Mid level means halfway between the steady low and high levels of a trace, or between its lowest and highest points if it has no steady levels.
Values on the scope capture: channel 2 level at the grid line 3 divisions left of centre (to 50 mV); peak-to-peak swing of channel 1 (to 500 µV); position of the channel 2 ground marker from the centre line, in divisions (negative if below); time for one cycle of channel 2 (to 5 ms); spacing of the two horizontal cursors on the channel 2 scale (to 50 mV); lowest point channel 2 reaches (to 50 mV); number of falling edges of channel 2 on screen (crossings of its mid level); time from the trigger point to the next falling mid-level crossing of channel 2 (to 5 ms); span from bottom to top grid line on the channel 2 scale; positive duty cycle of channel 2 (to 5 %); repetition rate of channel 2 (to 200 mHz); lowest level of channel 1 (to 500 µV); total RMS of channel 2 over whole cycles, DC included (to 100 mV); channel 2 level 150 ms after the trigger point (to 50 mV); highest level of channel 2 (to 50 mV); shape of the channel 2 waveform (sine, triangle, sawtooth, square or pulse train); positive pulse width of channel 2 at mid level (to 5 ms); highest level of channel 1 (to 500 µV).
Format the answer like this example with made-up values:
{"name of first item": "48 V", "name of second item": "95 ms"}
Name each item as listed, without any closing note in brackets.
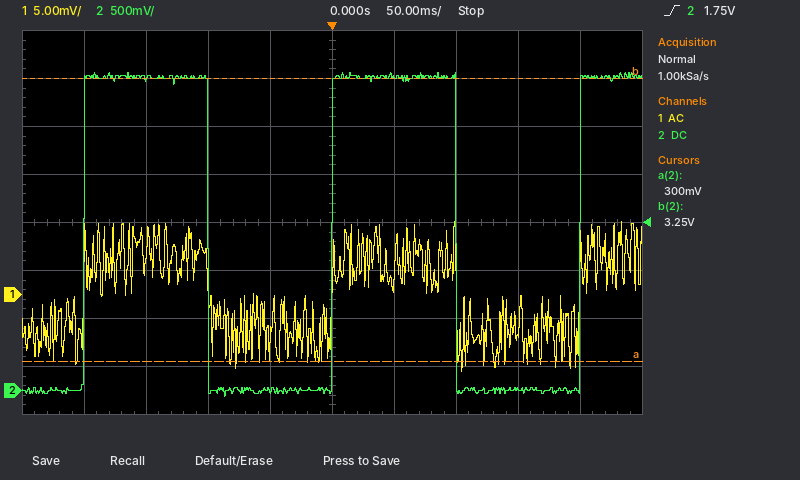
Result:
{"channel 2 level at the grid line 3 divisions left of centre": "3.25 V", "peak-to-peak swing of channel 1": "15.5 mV", "position of the channel 2 ground marker from the centre line, in divisions": "-3.5 div", "time for one cycle of channel 2": "200 ms", "spacing of the two horizontal cursors on the channel 2 scale": "2.95 V", "lowest point channel 2 reaches": "-50 mV", "number of falling edges of channel 2 on screen": "2", "time from the trigger point to the next falling mid-level crossing of channel 2": "100 ms", "span from bottom to top grid line on the channel 2 scale": "4 V", "positive duty cycle of channel 2": "50 %", "repetition rate of channel 2": "5.0 Hz", "lowest level of channel 1": "-8.0 mV", "total RMS of channel 2 over whole cycles, DC included": "2.3 V", "channel 2 level 150 ms after the trigger point": "0 mV", "highest level of channel 2": "3.30 V", "shape of the channel 2 waveform": "square", "positive pulse width of channel 2 at mid level": "100 ms", "highest level of channel 1": "7.5 mV"}
